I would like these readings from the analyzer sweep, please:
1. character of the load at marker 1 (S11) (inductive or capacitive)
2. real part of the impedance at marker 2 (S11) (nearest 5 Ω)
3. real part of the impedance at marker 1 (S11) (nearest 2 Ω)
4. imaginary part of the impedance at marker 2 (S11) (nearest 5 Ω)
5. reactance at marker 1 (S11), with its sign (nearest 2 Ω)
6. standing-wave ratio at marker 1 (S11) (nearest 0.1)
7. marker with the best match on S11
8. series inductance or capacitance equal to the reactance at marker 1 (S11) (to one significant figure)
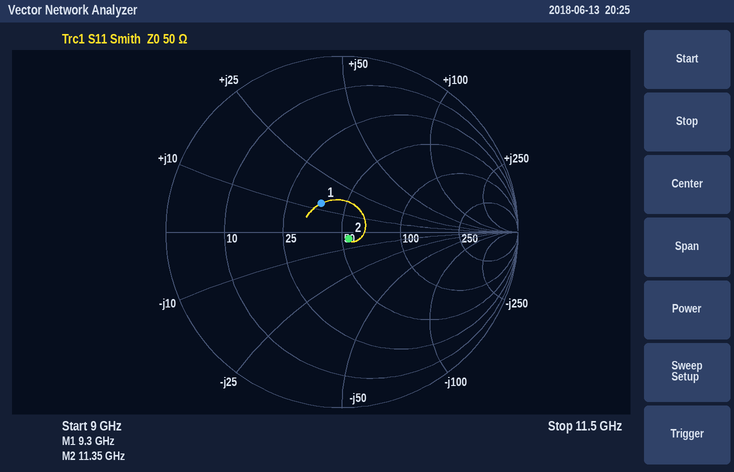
inductive
55 Ω
38 Ω
-5 Ω
+12 Ω
1.5
marker 2
200 pH
